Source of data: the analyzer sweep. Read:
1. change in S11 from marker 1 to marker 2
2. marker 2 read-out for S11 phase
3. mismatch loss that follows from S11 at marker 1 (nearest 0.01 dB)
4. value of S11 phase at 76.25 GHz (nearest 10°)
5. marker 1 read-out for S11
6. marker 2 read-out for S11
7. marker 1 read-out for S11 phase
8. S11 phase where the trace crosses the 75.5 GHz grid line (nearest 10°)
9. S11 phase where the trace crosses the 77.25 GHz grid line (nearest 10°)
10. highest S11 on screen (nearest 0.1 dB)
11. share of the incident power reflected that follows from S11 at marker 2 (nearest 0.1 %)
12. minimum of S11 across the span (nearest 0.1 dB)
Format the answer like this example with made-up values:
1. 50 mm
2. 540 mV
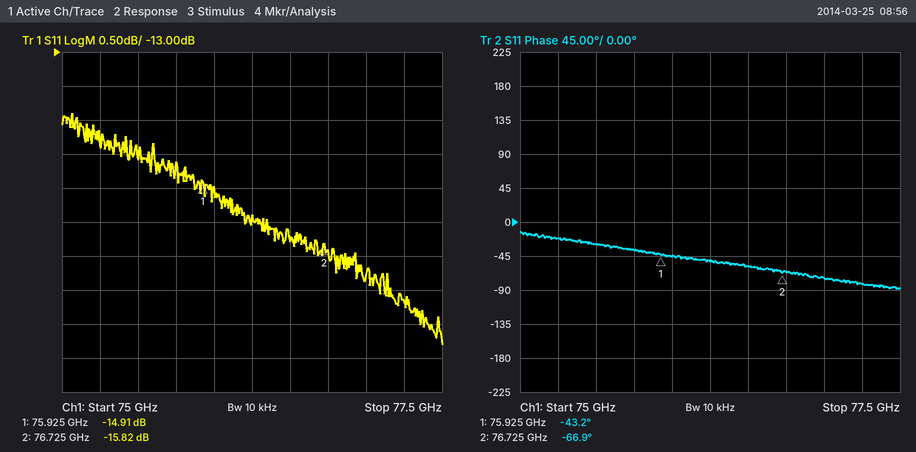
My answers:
1. -0.91 dB
2. -66.9°
3. 0.14 dB
4. -50°
5. -14.91 dB
6. -15.82 dB
7. -43.2°
8. -30°
9. -80°
10. -13.9 dB
11. 2.6 %
12. -17.3 dB
